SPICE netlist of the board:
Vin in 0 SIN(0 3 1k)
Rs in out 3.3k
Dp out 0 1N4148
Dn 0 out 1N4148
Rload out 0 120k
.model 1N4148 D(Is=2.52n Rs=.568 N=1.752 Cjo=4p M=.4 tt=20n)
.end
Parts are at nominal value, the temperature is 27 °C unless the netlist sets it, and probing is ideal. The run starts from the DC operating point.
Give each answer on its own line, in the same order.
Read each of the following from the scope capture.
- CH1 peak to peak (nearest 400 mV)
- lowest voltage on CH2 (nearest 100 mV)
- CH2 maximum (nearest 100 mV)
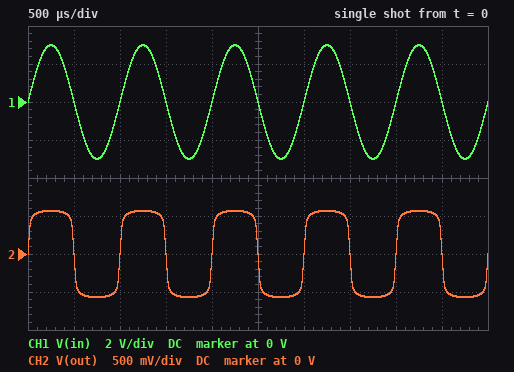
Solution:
6.0 V
-600 mV
600 mV
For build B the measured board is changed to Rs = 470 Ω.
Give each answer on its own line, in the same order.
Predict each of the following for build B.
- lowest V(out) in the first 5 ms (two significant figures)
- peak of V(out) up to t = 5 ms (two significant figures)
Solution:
-660 mV
660 mV
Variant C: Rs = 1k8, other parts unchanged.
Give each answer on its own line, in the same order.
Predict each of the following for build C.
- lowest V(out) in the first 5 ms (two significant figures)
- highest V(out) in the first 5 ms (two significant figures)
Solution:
-600 mV
600 mV
